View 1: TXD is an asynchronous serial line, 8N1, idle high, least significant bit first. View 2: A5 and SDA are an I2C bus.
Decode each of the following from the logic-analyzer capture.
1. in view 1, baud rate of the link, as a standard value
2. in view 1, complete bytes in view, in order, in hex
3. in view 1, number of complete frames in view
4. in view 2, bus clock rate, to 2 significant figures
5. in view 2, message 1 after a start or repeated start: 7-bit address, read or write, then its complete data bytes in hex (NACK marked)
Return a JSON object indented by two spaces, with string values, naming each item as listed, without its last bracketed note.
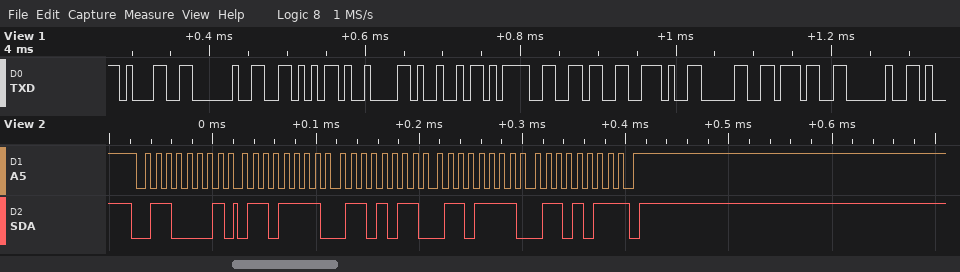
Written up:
{
  "in view 1, baud rate of the link, as a standard value": "115200 baud",
  "in view 1, complete bytes in view, in order, in hex": "31 20 56 09 49 3D 36 2E 30 37 20",
  "in view 1, number of complete frames in view": "11",
  "in view 2, bus clock rate, to 2 significant figures": "100 kHz",
  "in view 2, message 1 after a start or repeated start: 7-bit address, read or write, then its complete data bytes in hex": "0x30 read: 6F 6B 6F 6B NACK"
}
